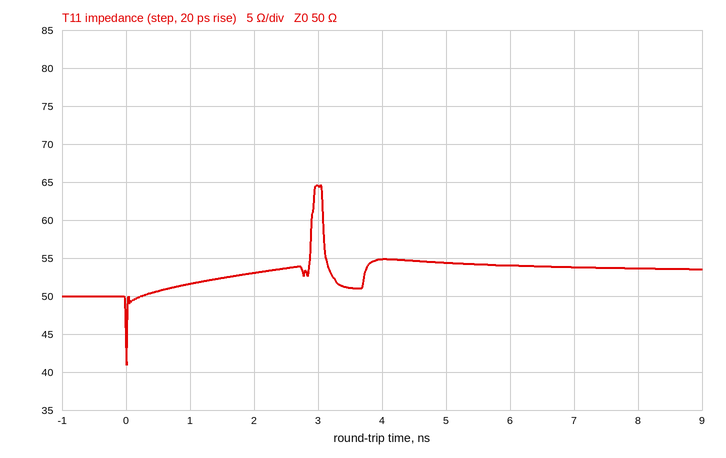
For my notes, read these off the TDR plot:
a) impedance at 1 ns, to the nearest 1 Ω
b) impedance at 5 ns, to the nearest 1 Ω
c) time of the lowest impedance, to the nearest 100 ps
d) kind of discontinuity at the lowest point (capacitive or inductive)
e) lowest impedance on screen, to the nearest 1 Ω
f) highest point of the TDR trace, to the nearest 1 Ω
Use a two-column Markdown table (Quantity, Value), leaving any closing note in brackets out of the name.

| Quantity | Value |
|---|---|
| impedance at 1 ns, to the nearest 1 Ω | 52 Ω |
| impedance at 5 ns, to the nearest 1 Ω | 54 Ω |
| time of the lowest impedance, to the nearest 100 ps | 0.0 ns |
| kind of discontinuity at the lowest point | capacitive |
| lowest impedance on screen, to the nearest 1 Ω | 41 Ω |
| highest point of the TDR trace, to the nearest 1 Ω | 65 Ω |
